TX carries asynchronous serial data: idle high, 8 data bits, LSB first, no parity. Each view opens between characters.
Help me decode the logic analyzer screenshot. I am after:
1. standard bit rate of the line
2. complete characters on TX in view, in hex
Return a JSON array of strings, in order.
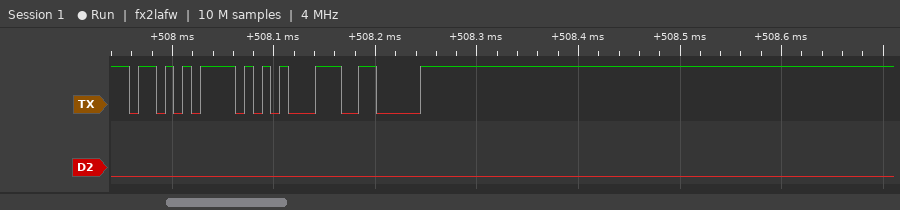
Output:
["115200 baud", "AB, 15, 06"]
